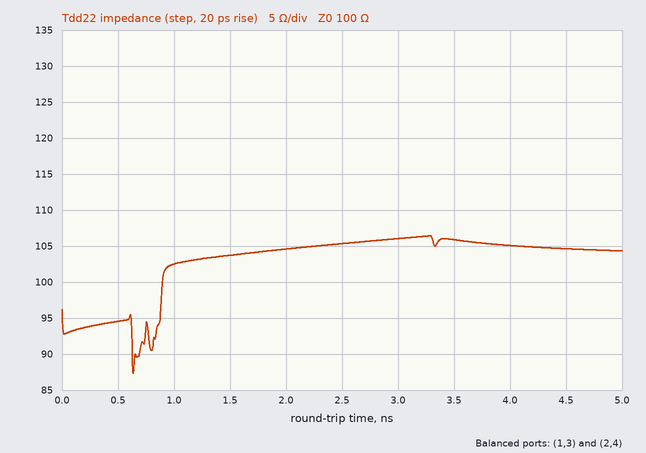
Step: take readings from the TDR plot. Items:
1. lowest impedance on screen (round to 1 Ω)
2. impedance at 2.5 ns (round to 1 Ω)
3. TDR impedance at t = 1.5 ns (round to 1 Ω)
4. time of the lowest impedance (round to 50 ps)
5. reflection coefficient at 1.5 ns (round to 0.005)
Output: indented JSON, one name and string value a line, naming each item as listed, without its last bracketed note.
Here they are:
{
  "lowest impedance on screen": "87 Ω",
  "impedance at 2.5 ns": "105 Ω",
  "TDR impedance at t = 1.5 ns": "104 Ω",
  "time of the lowest impedance": "650 ps",
  "reflection coefficient at 1.5 ns": "+0.020"
}
